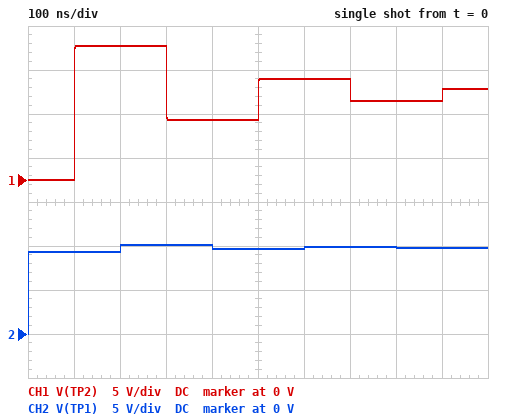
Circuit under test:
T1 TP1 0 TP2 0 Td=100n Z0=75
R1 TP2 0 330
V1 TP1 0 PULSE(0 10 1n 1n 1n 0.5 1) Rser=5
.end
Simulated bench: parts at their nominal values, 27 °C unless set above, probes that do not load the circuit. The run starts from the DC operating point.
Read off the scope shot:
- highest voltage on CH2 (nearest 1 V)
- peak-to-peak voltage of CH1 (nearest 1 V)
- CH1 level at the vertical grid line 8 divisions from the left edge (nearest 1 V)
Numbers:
10 V
15 V
9 V
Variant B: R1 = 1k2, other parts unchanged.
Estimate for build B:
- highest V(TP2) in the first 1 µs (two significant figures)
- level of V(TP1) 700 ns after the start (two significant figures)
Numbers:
18 V
10 V
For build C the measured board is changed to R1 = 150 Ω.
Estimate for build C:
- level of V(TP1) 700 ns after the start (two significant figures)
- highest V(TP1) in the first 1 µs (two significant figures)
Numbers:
9.7 V
9.8 V
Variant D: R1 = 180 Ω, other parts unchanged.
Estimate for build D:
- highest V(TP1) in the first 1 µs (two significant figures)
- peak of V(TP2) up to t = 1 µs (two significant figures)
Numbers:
9.9 V
13 V
